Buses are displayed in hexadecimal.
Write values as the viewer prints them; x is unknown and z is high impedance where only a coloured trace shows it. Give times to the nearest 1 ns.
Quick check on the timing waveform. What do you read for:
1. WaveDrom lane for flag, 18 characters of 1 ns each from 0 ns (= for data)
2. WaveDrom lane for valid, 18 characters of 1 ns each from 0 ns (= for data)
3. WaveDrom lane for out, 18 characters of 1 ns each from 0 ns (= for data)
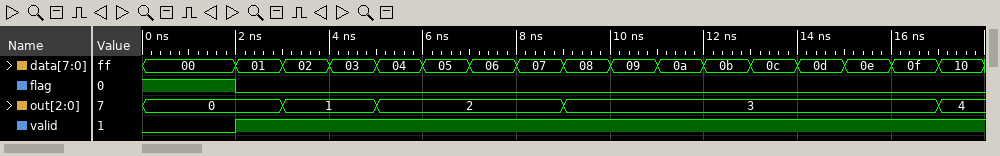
{name: 'flag', wave: '1.0...............'}
{name: 'valid', wave: '0.1...............'}
{name: 'out', wave: '=..=.=...=.......=', data: '0 1 2 3 4'}
